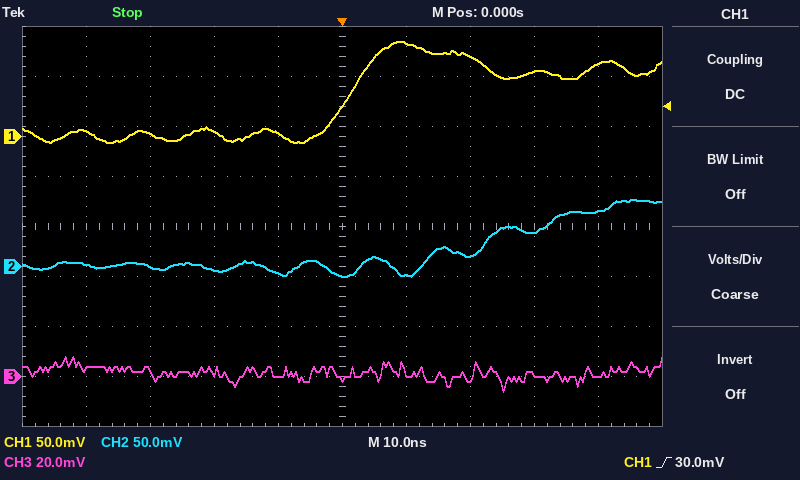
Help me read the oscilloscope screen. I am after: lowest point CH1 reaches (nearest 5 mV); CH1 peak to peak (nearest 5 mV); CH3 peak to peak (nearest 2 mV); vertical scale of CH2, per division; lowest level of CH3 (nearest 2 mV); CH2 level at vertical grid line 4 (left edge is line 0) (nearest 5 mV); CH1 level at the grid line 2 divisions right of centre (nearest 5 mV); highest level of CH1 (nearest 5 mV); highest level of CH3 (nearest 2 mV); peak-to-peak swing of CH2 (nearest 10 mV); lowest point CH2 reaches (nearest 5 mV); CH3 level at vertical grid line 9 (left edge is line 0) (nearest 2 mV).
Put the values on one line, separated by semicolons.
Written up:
-5 mV; 100 mV; 14 mV; 50 mV; -6 mV; -5 mV; 80 mV; 95 mV; 8 mV; 80 mV; -10 mV; 0 mV
